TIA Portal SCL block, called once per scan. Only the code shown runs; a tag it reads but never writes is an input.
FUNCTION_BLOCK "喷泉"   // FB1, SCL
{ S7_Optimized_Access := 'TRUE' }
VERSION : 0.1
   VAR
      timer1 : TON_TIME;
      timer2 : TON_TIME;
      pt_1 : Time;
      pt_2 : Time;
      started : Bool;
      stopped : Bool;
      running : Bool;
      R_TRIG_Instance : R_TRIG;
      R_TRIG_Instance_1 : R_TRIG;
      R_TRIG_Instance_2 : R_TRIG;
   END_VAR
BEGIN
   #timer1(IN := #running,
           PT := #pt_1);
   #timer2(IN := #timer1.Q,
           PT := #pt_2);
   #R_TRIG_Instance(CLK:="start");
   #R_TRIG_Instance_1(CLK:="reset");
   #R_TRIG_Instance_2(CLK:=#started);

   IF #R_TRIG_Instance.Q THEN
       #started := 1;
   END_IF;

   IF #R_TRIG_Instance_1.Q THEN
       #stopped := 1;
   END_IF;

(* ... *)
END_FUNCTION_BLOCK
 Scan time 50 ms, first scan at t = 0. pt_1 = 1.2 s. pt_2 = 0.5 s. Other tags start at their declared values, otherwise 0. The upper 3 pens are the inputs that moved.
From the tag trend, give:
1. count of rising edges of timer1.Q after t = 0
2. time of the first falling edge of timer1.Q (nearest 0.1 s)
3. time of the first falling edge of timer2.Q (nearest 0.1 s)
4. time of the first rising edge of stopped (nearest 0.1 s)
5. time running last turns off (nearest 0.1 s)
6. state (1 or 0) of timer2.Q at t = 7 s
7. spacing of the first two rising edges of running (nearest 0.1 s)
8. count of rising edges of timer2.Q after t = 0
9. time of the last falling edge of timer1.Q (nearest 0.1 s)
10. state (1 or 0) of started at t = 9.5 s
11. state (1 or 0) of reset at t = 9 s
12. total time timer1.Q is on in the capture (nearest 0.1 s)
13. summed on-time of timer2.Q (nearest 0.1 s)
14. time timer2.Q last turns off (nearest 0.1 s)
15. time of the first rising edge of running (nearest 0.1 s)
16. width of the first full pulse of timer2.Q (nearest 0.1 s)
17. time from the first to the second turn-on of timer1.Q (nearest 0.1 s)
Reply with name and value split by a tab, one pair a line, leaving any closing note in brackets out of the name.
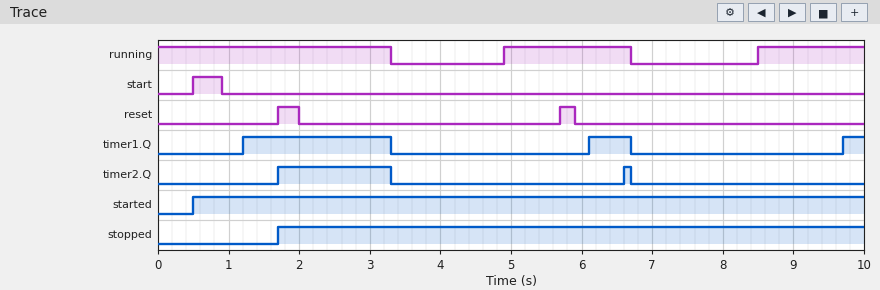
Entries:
count of rising edges of timer1.Q after t = 0	3
time of the first falling edge of timer1.Q	3.3 s
time of the first falling edge of timer2.Q	3.3 s
time of the first rising edge of stopped	1.7 s
time running last turns off	6.7 s
state (1 or 0) of timer2.Q at t = 7 s	0
spacing of the first two rising edges of running	3.6 s
count of rising edges of timer2.Q after t = 0	2
time of the last falling edge of timer1.Q	6.7 s
state (1 or 0) of started at t = 9.5 s	1
state (1 or 0) of reset at t = 9 s	0
total time timer1.Q is on in the capture	3.0 s
summed on-time of timer2.Q	1.7 s
time timer2.Q last turns off	6.7 s
time of the first rising edge of running	4.9 s
width of the first full pulse of timer2.Q	1.6 s
time from the first to the second turn-on of timer1.Q	4.9 s
